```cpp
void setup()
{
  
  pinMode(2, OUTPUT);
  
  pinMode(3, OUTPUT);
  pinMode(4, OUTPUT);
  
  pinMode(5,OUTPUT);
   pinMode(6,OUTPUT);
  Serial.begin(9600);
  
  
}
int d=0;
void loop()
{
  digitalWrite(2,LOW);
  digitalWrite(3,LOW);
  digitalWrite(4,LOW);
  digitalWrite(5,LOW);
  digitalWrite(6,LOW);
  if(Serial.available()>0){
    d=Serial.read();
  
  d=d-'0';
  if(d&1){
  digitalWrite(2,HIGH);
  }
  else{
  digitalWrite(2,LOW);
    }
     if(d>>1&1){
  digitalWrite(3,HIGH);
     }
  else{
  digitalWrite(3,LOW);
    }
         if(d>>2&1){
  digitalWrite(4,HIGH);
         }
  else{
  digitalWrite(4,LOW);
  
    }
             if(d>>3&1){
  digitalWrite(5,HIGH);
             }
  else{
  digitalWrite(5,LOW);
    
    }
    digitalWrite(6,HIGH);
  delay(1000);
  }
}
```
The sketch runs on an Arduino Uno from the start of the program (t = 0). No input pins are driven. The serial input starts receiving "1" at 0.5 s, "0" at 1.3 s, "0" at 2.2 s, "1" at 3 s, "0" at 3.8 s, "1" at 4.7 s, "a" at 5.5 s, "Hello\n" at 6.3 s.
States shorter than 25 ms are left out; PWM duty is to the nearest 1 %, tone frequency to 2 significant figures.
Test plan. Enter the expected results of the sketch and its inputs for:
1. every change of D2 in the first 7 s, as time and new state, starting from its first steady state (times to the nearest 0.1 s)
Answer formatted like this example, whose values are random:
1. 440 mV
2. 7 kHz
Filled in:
1. 0 s low; 0.5 s high; 1.5 s low; 3.5 s high; 4.5 s low; 5.5 s high
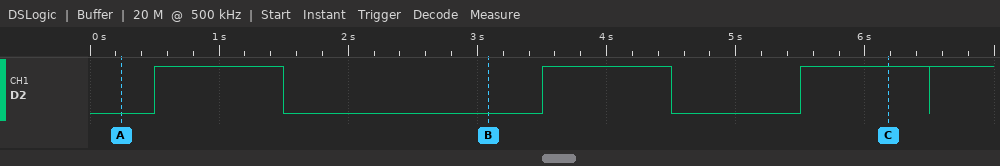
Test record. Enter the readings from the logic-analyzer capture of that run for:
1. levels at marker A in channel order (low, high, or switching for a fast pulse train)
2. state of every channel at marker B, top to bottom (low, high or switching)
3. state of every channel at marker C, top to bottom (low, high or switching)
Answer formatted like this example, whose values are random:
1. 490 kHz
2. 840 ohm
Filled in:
1. D2 low
2. D2 low
3. D2 high
